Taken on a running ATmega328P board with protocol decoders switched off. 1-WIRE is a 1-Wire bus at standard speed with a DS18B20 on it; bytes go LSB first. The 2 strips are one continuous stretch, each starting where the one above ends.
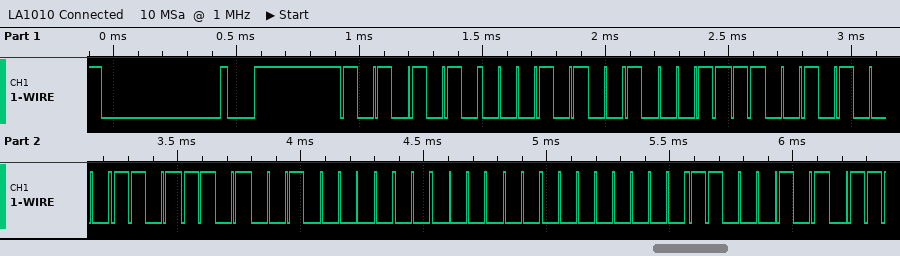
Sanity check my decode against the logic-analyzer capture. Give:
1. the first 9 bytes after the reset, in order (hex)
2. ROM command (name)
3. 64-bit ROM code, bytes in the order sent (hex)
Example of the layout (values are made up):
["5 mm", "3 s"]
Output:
["55 28 F1 14 BB 04 00 00 A3", "Match ROM", "28 F1 14 BB 04 00 00 A3"]
